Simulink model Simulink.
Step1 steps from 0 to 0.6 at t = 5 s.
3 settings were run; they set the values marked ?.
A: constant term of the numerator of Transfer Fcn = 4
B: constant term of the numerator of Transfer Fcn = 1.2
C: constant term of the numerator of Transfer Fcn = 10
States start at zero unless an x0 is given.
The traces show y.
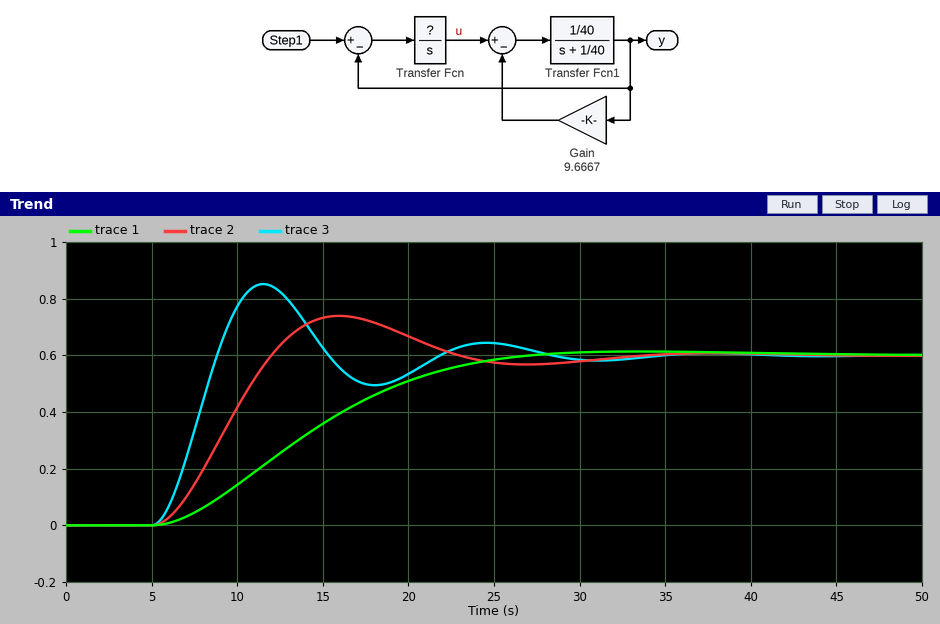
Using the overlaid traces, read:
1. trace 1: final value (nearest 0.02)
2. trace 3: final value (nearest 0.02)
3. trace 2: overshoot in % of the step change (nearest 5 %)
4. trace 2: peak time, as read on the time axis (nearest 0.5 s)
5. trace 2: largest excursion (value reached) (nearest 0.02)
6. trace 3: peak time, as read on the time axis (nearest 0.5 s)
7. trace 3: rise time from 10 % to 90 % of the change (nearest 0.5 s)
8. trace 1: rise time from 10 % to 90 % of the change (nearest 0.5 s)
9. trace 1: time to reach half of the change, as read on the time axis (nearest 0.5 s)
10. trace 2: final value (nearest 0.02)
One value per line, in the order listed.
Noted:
0.60
0.60
25 %
16.0 s
0.74
11.5 s
2.5 s
13.5 s
13.5 s
0.60
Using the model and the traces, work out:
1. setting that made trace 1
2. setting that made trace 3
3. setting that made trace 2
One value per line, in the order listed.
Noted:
B
C
A
